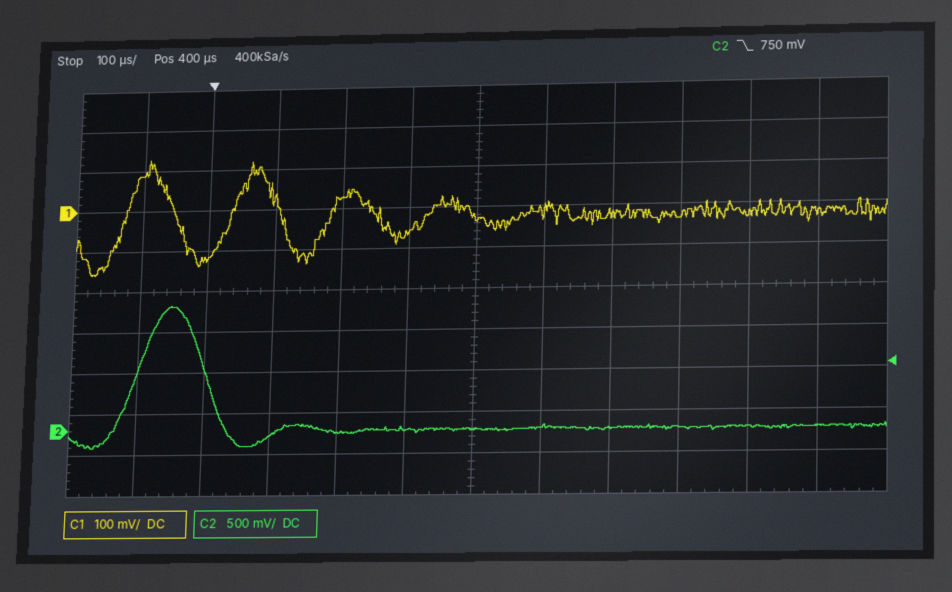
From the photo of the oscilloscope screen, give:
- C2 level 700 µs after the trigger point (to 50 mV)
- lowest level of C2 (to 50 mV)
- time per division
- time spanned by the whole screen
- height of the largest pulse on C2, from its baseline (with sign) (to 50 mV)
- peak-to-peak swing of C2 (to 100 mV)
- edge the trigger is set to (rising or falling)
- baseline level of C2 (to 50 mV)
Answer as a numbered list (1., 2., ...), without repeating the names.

1. 0 mV
2. -200 mV
3. 100 µs
4. 1.2 ms
5. +1.55 V
6. 1.70 V
7. falling
8. 0 mV
